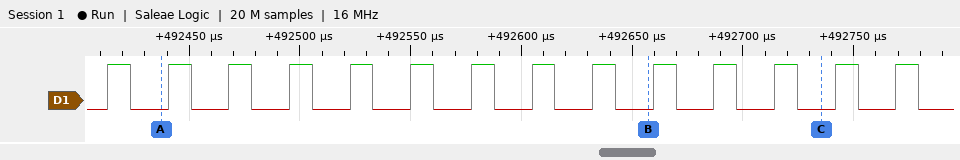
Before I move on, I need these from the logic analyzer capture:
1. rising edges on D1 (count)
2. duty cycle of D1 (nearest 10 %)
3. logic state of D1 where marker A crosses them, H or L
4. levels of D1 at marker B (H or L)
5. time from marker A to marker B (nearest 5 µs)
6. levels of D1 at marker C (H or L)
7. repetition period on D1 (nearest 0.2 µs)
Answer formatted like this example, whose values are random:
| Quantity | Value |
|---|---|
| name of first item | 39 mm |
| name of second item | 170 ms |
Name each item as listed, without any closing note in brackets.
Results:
| Quantity | Value |
|---|---|
| rising edges on D1 | 14 |
| duty cycle of D1 | 40 % |
| logic state of D1 where marker A crosses them, H or L | D1=L |
| levels of D1 at marker B | D1=L |
| time from marker A to marker B | 220 µs |
| levels of D1 at marker C | D1=L |
| repetition period on D1 | 27.4 µs |
